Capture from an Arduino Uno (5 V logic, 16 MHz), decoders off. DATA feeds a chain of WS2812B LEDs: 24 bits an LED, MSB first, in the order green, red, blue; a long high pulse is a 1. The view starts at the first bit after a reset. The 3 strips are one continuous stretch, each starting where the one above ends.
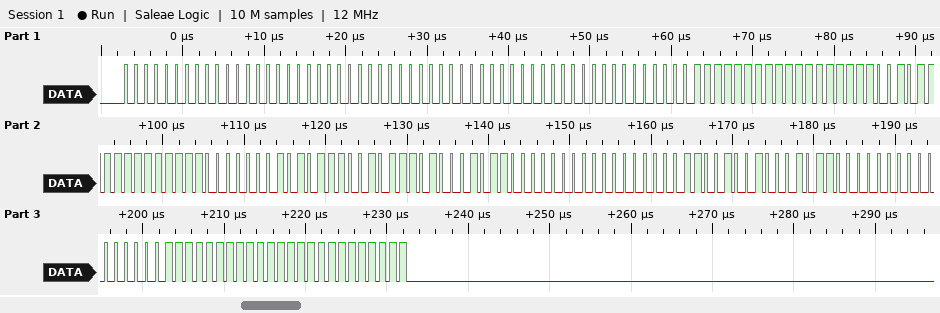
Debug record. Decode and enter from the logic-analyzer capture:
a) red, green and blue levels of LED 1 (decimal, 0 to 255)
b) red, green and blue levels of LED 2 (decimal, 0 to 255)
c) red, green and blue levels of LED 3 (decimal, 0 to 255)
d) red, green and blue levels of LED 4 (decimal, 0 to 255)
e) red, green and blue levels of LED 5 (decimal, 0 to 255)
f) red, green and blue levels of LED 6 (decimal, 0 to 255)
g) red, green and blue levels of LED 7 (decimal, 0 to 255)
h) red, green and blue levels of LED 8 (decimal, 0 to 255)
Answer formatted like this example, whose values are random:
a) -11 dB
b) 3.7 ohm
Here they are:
a) 0, 0, 0
b) 0, 0, 0
c) 255, 0, 255
d) 255, 203, 192
e) 46, 87, 139
f) 0, 0, 100
g) 0, 139, 0
h) 255, 255, 255
